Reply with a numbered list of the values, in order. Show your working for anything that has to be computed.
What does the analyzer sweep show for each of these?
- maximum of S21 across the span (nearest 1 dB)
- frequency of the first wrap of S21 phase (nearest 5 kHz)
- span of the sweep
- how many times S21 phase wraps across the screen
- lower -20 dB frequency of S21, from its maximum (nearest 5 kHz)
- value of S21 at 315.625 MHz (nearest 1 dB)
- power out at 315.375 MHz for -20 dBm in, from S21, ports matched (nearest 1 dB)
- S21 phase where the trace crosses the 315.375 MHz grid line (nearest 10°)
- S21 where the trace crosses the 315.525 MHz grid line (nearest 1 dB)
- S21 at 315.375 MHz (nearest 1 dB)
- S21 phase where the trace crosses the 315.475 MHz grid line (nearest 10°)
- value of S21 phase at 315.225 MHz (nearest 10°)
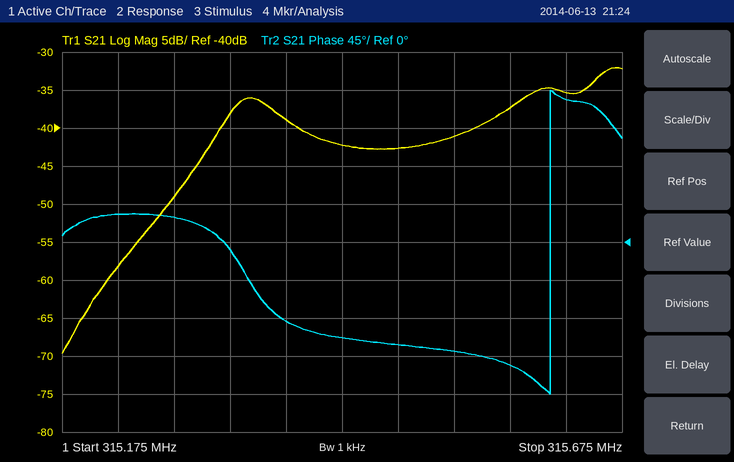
1. -32 dB
2. 315.610 MHz
3. 500 kHz
4. 1
5. 315.260 MHz
6. -35 dB
7. -20 dBm + (-39 dB) = -59 dBm
8. -90°
9. -41 dB
10. -39 dB
11. -120°
12. 30°
